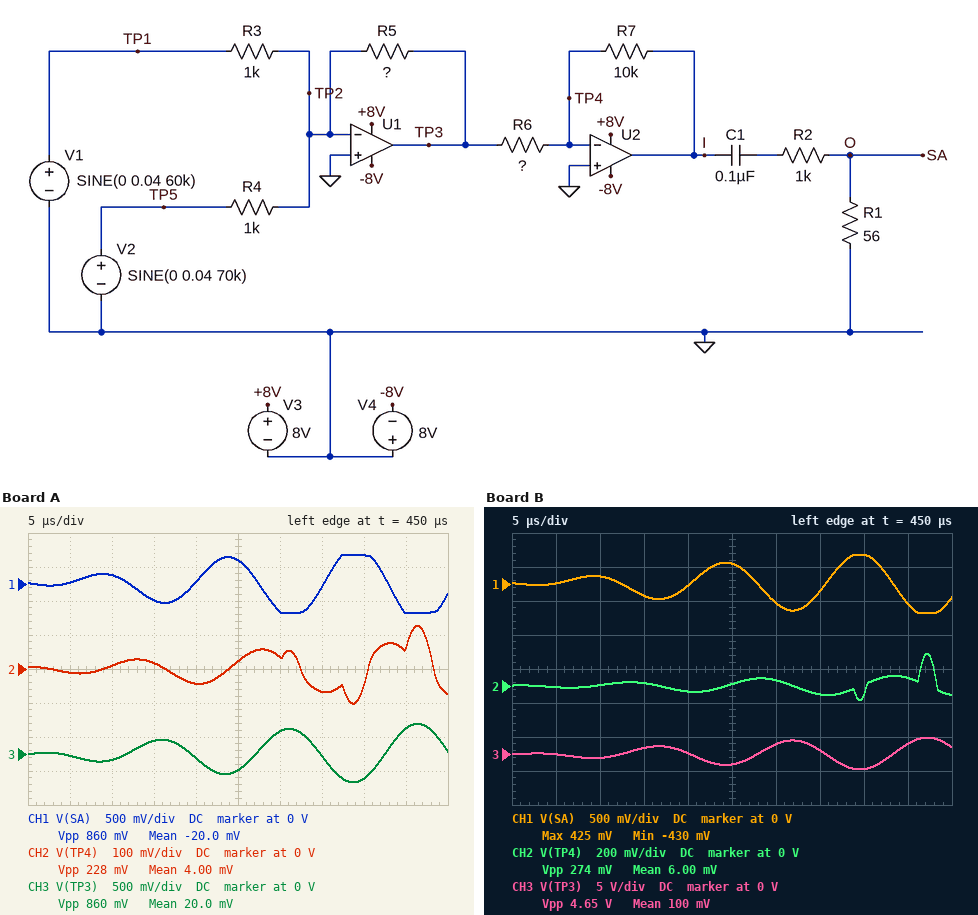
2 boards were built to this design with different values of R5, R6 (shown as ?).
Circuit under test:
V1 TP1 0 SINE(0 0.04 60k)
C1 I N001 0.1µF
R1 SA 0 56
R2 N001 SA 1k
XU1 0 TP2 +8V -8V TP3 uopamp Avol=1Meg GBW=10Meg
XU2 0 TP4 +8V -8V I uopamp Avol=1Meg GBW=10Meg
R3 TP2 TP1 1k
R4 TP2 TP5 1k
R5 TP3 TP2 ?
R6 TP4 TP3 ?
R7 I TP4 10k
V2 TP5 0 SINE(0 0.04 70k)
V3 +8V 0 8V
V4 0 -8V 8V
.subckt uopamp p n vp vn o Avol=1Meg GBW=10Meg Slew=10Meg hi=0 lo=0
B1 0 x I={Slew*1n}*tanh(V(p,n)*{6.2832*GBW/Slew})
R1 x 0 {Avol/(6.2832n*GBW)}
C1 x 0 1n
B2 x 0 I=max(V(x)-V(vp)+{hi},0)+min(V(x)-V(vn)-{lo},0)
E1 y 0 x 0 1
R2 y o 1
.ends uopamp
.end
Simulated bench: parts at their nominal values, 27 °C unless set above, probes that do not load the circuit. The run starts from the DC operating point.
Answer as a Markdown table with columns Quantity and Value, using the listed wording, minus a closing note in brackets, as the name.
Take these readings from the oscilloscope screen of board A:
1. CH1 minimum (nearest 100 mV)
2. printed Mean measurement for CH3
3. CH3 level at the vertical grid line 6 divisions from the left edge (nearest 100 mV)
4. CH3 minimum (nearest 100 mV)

| Quantity | Value |
|---|---|
| CH1 minimum | -400 mV |
| printed Mean measurement for CH3 | 20.0 mV |
| CH3 level at the vertical grid line 6 divisions from the left edge | 300 mV |
| CH3 minimum | -400 mV |
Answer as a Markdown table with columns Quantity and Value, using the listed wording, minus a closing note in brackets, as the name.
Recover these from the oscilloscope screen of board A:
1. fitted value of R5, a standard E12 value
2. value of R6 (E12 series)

| Quantity | Value |
|---|---|
| fitted value of R5, a standard E12 value | 5.6 kΩ |
| value of R6 | 390 Ω |
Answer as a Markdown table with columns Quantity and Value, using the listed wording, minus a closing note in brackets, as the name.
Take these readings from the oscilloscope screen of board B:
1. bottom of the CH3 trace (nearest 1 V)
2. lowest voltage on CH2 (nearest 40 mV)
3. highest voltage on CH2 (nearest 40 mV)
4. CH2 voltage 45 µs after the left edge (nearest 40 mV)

| Quantity | Value |
|---|---|
| bottom of the CH3 trace | -2 V |
| lowest voltage on CH2 | -80 mV |
| highest voltage on CH2 | 200 mV |
| CH2 voltage 45 µs after the left edge | 40 mV |
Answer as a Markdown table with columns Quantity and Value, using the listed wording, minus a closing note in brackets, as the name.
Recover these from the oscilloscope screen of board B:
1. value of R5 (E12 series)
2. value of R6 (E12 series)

| Quantity | Value |
|---|---|
| value of R5 | 33 kΩ |
| value of R6 | 2.7 kΩ |
